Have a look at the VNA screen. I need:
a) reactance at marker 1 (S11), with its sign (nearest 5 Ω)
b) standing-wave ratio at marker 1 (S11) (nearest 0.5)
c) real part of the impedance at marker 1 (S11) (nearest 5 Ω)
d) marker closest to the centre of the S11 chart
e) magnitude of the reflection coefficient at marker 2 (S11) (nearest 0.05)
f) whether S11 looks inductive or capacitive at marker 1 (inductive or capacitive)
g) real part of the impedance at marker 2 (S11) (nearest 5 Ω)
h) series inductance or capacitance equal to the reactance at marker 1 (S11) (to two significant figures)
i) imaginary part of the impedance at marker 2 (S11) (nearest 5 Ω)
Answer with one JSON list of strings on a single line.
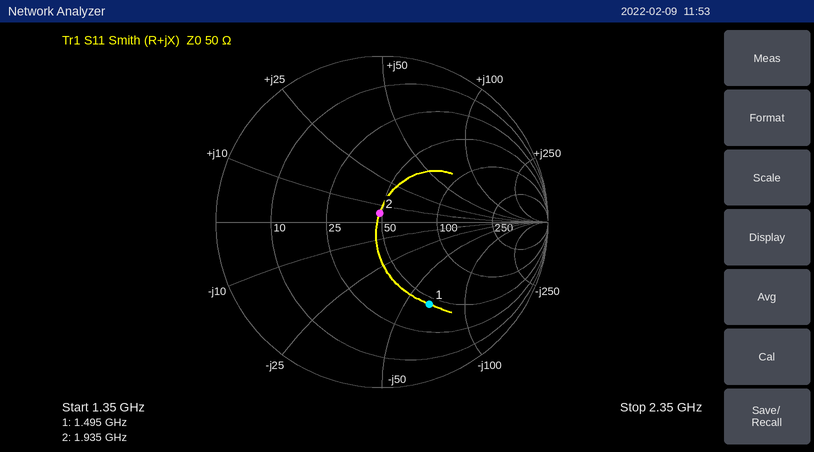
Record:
["-65 Ω", "3.5", "45 Ω", "marker 2", "0.05", "capacitive", "50 Ω", "1.6 pF", "+5 Ω"]
